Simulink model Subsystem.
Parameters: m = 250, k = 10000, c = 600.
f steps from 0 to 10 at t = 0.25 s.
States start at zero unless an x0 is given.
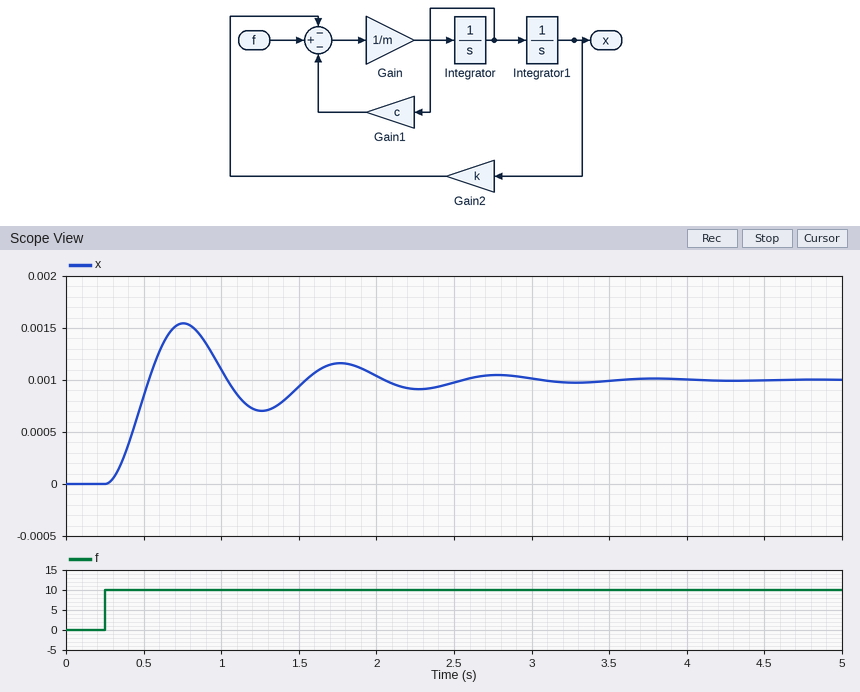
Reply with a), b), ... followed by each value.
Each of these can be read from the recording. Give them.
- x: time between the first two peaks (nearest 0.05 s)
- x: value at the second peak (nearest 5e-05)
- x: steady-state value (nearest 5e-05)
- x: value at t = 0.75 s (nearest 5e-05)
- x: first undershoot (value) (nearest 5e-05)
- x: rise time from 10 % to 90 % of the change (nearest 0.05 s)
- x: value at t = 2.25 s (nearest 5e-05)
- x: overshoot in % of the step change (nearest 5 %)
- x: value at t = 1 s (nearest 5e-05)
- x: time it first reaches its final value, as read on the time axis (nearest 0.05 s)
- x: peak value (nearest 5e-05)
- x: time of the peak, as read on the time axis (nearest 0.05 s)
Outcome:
a) 1.00 s
b) 0.00115
c) 0.00100
d) 0.00155
e) 0.00070
f) 0.20 s
g) 0.00090
h) 55 %
i) 0.00110
j) 0.55 s
k) 0.00155
l) 0.75 s
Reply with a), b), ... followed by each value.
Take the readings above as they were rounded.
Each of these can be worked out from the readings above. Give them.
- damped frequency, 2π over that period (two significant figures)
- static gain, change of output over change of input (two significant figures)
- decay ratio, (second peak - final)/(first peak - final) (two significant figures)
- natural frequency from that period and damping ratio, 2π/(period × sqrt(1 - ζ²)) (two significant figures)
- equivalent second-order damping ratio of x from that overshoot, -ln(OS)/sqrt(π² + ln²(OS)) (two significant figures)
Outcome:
a) 6.3 rad/s
b) 0.00010
c) 0.27
d) 6.4 rad/s
e) 0.19
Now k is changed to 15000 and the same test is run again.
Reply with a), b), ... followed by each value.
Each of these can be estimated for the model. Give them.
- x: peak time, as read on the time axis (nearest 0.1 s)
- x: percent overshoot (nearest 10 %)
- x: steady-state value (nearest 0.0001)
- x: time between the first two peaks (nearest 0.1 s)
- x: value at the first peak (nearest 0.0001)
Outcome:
a) 0.7 s
b) 60 %
c) 0.0007
d) 0.8 s
e) 0.0011
